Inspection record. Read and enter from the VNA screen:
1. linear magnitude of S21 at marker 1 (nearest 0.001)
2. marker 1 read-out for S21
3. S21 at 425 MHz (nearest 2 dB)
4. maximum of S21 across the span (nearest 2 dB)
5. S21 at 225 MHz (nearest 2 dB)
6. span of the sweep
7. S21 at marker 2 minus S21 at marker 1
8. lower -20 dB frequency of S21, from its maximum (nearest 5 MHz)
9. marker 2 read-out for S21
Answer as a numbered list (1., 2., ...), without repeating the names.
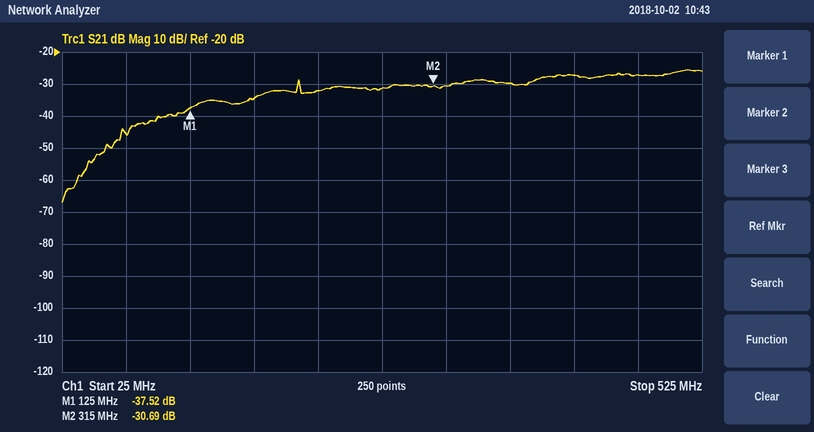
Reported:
1. 0.013
2. -37.52 dB
3. -28 dB
4. -26 dB
5. -32 dB
6. 500 MHz
7. 6.83 dB
8. 75 MHz
9. -30.69 dB
